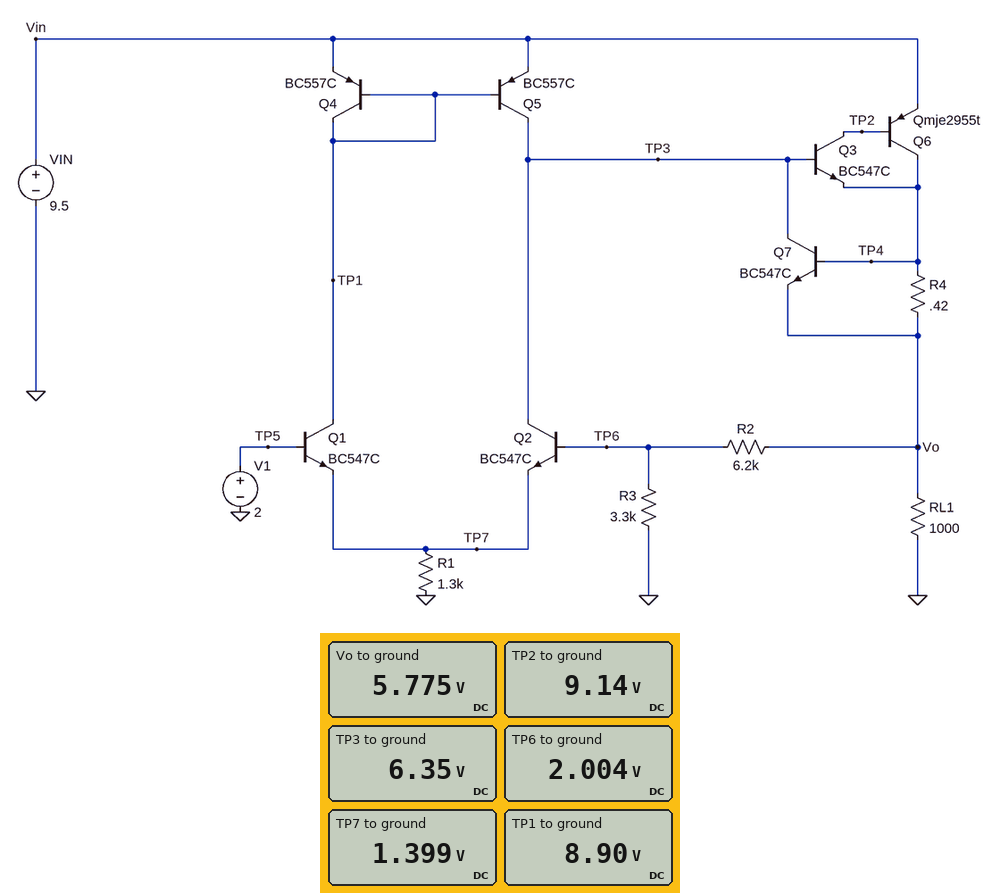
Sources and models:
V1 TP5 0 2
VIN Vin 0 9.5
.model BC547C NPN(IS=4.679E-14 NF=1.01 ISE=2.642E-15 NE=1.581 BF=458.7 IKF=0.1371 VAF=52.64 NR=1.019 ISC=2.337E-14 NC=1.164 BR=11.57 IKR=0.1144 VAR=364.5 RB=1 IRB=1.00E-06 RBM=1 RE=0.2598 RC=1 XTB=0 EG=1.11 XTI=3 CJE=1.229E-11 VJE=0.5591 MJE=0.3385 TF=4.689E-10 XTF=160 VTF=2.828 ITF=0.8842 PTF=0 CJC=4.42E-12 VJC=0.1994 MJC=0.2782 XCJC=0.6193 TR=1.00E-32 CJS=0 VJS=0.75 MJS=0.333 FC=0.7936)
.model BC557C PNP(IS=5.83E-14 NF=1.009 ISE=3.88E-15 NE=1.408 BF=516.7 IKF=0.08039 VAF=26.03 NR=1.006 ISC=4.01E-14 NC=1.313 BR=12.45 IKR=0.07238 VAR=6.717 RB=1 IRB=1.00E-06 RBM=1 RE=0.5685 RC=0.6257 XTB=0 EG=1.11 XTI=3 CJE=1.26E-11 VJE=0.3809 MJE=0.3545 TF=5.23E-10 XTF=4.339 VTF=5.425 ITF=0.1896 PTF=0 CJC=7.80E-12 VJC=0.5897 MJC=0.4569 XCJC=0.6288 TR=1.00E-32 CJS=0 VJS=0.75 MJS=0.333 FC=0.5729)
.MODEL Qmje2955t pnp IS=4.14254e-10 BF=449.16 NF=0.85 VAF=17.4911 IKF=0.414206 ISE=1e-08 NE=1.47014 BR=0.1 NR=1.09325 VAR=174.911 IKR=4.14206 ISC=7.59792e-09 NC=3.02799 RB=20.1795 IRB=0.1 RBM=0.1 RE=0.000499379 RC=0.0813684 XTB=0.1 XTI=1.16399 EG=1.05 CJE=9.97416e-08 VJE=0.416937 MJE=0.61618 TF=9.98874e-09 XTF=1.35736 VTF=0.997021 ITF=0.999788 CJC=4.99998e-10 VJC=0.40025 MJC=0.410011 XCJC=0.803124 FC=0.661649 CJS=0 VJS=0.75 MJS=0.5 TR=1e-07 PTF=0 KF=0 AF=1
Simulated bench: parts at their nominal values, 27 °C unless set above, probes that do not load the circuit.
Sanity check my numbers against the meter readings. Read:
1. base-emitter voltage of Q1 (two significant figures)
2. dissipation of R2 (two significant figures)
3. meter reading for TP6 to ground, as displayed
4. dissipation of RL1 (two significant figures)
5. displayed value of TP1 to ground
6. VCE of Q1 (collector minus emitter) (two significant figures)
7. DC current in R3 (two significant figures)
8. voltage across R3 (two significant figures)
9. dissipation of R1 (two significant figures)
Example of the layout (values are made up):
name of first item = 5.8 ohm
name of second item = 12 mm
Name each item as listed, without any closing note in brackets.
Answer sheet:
base-emitter voltage of Q1 = 600 mV
dissipation of R2 = 2.3 mW
meter reading for TP6 to ground, as displayed = 2.004 V
dissipation of RL1 = 33 mW
displayed value of TP1 to ground = 8.90 V
VCE of Q1 (collector minus emitter) = 7.5 V
DC current in R3 = 610 µA
voltage across R3 = 2.0 V
dissipation of R1 = 1.5 mW
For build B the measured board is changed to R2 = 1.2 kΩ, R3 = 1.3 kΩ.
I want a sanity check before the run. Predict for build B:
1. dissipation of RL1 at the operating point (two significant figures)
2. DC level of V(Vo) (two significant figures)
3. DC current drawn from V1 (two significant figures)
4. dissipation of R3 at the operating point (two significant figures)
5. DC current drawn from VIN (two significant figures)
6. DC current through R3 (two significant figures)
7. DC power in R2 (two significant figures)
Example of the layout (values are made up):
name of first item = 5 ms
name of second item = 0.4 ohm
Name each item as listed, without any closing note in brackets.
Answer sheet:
dissipation of RL1 at the operating point = 15 mW
DC level of V(Vo) = 3.9 V
DC current drawn from V1 = 960 nA
dissipation of R3 at the operating point = 3.1 mW
DC current drawn from VIN = 6.5 mA
DC current through R3 = 1.5 mA
DC power in R2 = 2.9 mW
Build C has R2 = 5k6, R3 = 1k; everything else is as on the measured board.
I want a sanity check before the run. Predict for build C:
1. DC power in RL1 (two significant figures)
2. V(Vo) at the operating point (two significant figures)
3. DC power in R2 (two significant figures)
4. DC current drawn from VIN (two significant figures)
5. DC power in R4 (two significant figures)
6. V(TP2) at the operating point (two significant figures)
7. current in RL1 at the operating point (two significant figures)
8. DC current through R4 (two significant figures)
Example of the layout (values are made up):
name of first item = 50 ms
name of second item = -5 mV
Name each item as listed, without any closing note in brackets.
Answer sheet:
DC power in RL1 = 79 mW
V(Vo) at the operating point = 8.9 V
DC power in R2 = 10 mW
DC current drawn from VIN = 11 mA
DC power in R4 = 44 µW
V(TP2) at the operating point = 9.1 V
current in RL1 at the operating point = 8.9 mA
DC current through R4 = 10 mA
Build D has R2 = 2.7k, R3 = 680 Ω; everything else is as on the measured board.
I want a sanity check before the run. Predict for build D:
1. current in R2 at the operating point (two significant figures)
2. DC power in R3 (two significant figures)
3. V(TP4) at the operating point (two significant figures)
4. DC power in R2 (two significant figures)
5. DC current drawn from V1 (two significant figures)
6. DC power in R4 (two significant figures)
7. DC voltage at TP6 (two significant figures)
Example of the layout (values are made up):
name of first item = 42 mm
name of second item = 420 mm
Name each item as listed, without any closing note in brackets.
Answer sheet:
current in R2 at the operating point = 2.6 mA
DC power in R3 = 4.7 mW
V(TP4) at the operating point = 8.9 V
DC power in R2 = 19 mW
DC current drawn from V1 = 2.1 µA
DC power in R4 = 56 µW
DC voltage at TP6 = 1.8 V
